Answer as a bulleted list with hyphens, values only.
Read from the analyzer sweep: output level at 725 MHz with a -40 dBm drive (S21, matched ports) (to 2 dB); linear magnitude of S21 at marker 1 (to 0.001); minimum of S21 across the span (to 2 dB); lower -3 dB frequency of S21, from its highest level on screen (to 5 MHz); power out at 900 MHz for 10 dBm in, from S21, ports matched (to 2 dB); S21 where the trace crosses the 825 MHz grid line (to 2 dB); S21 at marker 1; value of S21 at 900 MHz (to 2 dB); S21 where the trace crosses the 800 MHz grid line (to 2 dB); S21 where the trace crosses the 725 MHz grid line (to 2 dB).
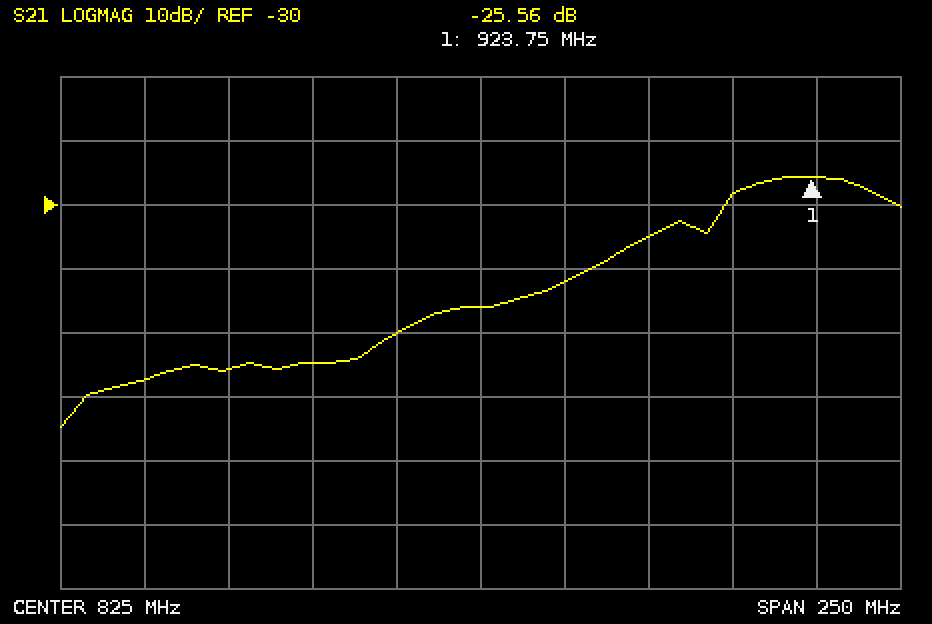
- -98 dBm
- 0.053
- -64 dB
- 900 MHz
- -18 dBm
- -46 dB
- -25.56 dB
- -28 dB
- -50 dB
- -58 dB
